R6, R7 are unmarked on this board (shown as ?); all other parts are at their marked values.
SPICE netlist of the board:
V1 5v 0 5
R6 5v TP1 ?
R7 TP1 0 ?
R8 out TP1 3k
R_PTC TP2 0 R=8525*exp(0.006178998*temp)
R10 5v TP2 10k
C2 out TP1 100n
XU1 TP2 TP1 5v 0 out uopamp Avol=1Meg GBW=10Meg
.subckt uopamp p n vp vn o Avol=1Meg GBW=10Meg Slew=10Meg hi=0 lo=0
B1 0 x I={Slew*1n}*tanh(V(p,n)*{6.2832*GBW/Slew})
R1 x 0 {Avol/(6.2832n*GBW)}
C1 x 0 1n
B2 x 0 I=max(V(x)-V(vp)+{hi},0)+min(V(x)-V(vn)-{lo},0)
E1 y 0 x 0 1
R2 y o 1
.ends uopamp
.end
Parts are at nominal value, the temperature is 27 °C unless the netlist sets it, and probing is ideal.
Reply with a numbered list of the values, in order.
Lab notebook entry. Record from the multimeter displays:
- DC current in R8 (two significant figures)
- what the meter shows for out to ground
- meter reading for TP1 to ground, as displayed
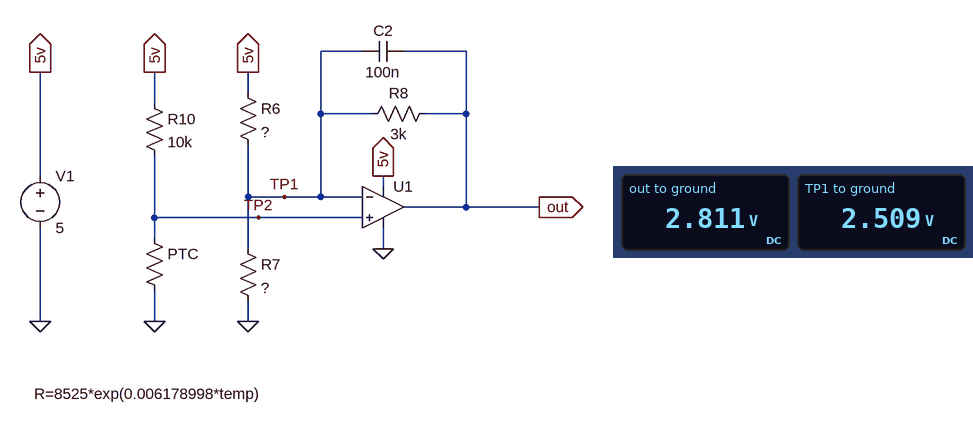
1. 100 µA
2. 2.811 V
3. 2.509 V
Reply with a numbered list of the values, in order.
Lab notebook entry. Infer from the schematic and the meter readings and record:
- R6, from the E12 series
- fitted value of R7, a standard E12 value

1. 180 Ω
2. 180 Ω
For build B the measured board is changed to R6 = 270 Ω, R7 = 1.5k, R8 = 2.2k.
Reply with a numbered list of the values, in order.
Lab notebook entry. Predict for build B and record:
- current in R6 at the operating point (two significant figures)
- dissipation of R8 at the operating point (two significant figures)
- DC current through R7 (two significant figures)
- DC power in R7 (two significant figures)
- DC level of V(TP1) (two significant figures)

1. 4.3 mA
2. 6.7 mW
3. 2.6 mA
4. 9.8 mW
5. 3.8 V
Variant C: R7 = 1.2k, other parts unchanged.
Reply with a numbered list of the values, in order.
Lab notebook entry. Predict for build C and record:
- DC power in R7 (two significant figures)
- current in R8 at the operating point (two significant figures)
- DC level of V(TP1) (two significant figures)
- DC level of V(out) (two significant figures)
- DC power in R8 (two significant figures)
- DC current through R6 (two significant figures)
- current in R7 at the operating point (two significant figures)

1. 14 mW
2. 1.4 mA
3. 4.1 V
4. -8.6 mV
5. 5.7 mW
6. 4.8 mA
7. 3.4 mA
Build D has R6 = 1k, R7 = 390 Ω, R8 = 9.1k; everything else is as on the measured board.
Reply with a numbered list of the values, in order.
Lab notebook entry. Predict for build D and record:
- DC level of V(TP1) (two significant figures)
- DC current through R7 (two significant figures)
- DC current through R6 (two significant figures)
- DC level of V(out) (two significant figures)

1. 1.5 V
2. 3.9 mA
3. 3.5 mA
4. 5.0 V
